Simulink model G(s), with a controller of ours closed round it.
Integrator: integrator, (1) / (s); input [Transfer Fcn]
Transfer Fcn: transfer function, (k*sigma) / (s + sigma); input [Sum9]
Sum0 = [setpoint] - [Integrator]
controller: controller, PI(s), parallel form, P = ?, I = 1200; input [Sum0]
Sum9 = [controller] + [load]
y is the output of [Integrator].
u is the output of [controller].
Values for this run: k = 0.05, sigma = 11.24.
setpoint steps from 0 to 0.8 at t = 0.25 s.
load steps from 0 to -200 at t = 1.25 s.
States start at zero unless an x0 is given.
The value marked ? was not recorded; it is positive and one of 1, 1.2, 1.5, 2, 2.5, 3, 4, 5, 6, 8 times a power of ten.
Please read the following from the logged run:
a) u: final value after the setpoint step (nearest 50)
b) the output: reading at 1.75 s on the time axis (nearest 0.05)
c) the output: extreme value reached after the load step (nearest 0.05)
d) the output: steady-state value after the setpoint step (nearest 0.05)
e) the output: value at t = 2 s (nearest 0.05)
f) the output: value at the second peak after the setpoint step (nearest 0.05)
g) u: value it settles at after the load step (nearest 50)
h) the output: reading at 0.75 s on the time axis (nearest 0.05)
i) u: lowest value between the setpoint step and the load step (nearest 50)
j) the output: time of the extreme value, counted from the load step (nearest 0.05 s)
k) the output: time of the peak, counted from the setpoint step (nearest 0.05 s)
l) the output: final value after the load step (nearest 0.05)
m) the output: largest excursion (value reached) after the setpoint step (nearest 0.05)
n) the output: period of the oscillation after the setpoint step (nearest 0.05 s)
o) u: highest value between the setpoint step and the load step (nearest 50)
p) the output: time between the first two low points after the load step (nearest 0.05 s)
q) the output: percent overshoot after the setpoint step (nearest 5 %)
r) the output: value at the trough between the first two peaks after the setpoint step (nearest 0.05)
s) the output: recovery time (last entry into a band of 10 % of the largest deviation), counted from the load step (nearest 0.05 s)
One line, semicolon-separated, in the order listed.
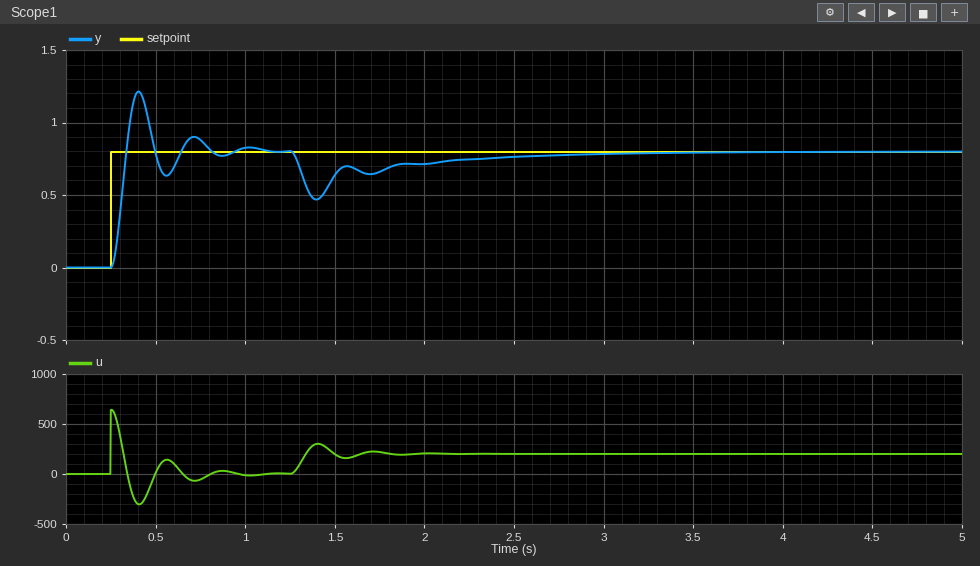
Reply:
0; 0.65; 0.45; 0.80; 0.70; 0.90; 200; 0.90; -300; 0.15 s; 0.15 s; 0.80; 1.20; 0.30 s; 650; 0.30 s; 50 %; 0.65; 1.35 s
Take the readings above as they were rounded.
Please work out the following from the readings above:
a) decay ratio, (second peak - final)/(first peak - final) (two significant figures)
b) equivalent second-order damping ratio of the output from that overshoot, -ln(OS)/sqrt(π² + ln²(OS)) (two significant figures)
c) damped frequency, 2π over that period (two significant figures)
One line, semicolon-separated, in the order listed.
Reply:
0.25; 0.22; 21 rad/s
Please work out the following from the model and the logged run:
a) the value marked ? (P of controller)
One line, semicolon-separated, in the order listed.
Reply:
800
